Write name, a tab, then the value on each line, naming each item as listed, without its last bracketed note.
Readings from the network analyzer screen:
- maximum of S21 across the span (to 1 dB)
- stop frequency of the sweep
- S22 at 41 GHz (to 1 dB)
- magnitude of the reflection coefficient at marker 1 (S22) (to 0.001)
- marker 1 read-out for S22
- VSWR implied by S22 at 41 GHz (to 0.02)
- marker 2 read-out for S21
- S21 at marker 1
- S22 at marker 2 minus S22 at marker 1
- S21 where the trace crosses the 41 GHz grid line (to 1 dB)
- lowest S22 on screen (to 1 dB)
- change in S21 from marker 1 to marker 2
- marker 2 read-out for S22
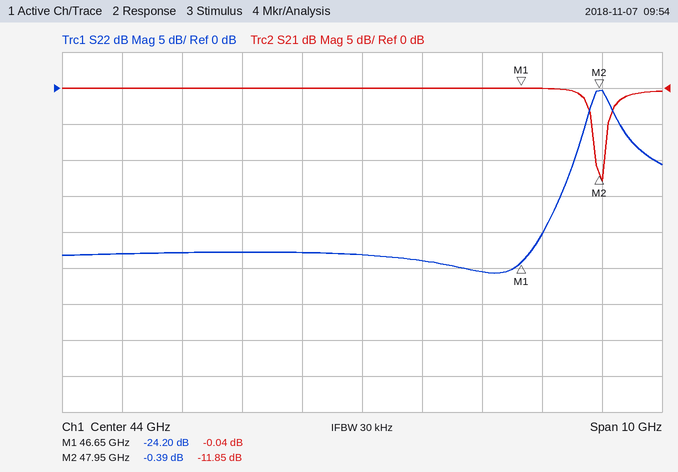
maximum of S21 across the span	0 dB
stop frequency of the sweep	49 GHz
S22 at 41 GHz	-23 dB
magnitude of the reflection coefficient at marker 1 (S22)	0.062
marker 1 read-out for S22	-24.20 dB
VSWR implied by S22 at 41 GHz	1.16
marker 2 read-out for S21	-11.85 dB
S21 at marker 1	-0.04 dB
S22 at marker 2 minus S22 at marker 1	23.81 dB
S21 where the trace crosses the 41 GHz grid line	0 dB
lowest S22 on screen	-26 dB
change in S21 from marker 1 to marker 2	-11.81 dB
marker 2 read-out for S22	-0.39 dB
